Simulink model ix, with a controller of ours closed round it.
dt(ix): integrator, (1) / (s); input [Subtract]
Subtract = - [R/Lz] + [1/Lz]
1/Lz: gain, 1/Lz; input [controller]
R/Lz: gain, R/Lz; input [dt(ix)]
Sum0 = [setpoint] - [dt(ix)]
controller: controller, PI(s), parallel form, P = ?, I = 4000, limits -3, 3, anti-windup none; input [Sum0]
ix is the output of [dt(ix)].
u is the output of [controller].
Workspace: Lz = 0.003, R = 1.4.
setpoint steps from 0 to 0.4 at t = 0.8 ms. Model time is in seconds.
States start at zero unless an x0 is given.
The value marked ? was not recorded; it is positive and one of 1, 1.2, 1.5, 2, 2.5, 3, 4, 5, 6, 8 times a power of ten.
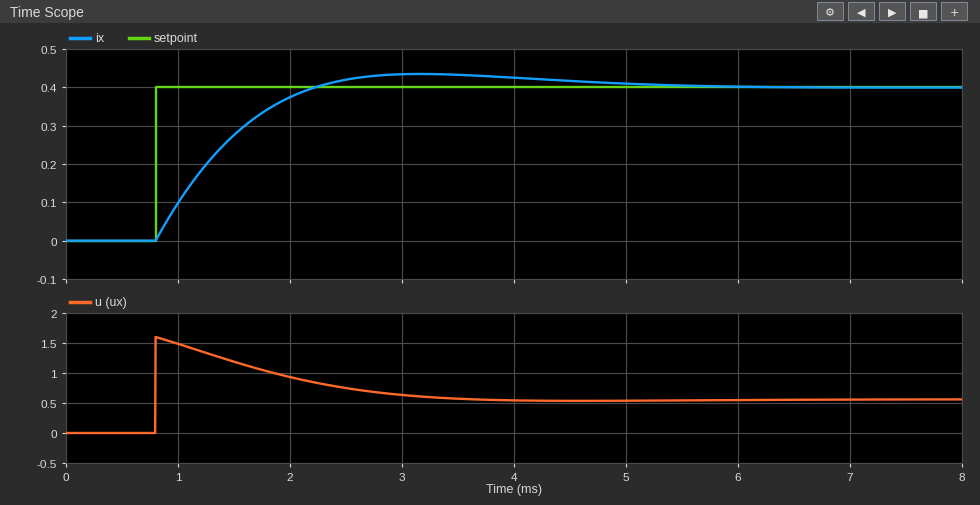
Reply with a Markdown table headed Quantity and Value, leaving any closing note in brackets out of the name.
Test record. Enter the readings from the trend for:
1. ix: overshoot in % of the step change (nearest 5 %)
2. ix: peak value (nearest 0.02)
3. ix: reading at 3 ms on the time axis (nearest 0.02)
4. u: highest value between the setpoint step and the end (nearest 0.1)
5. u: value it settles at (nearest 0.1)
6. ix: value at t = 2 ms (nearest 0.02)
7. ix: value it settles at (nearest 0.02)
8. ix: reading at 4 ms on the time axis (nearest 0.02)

| Quantity | Value |
|---|---|
| ix: overshoot in % of the step change | 10 % |
| ix: peak value | 0.44 |
| ix: reading at 3 ms on the time axis | 0.44 |
| u: highest value between the setpoint step and the end | 1.6 |
| u: value it settles at | 0.6 |
| ix: value at t = 2 ms | 0.38 |
| ix: value it settles at | 0.40 |
| ix: reading at 4 ms on the time axis | 0.42 |
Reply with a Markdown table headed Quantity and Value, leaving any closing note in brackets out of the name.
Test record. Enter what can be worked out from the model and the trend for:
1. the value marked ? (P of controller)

| Quantity | Value |
|---|---|
| the value marked ? | 4 |
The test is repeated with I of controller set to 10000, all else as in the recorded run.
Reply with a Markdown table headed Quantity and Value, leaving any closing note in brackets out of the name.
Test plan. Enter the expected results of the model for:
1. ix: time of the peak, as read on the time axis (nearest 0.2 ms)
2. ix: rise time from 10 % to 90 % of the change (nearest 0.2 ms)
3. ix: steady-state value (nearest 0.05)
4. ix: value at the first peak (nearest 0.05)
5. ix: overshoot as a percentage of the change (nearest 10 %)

| Quantity | Value |
|---|---|
| ix: time of the peak, as read on the time axis | 2.2 ms |
| ix: rise time from 10 % to 90 % of the change | 0.6 ms |
| ix: steady-state value | 0.40 |
| ix: value at the first peak | 0.50 |
| ix: overshoot as a percentage of the change | 20 % |
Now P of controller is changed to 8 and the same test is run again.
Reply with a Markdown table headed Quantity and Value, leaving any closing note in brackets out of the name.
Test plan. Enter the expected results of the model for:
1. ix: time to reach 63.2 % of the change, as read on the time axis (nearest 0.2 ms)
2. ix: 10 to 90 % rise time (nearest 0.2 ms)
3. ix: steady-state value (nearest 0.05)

| Quantity | Value |
|---|---|
| ix: time to reach 63.2 % of the change, as read on the time axis | 1.2 ms |
| ix: 10 to 90 % rise time | 0.8 ms |
| ix: steady-state value | 0.40 |
